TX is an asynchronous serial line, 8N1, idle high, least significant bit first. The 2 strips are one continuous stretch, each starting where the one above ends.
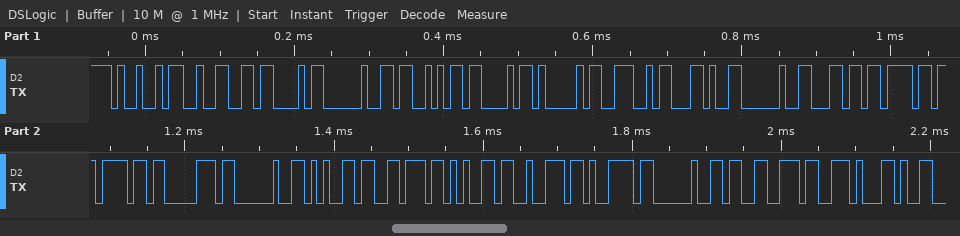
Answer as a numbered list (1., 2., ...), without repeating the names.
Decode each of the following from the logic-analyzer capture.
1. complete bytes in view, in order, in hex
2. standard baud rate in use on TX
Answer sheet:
1. 49 32 43 20 53 43 41 4E 2C 20 6C 6F 6F 70 20 65 76 65 72 79 20 33 73 2C
2. 115200 baud
